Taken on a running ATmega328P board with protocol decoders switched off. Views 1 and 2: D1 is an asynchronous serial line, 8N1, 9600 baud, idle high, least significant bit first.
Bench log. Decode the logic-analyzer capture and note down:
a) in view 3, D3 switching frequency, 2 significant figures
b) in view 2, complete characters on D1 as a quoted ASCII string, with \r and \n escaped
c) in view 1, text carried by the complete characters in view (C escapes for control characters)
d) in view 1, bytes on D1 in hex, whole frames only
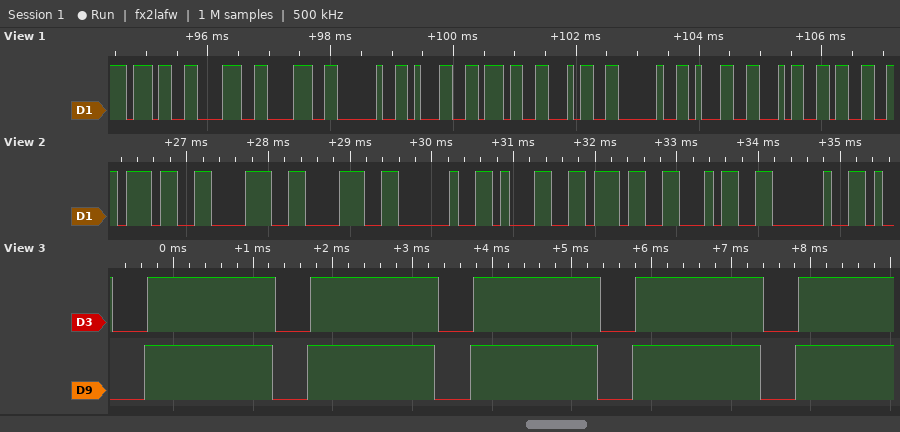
490 Hz
"788 174 "
"788 174 143"
0x37 0x38 0x38 0x20 0x31 0x37 0x34 0x20 0x31 0x34 0x33
